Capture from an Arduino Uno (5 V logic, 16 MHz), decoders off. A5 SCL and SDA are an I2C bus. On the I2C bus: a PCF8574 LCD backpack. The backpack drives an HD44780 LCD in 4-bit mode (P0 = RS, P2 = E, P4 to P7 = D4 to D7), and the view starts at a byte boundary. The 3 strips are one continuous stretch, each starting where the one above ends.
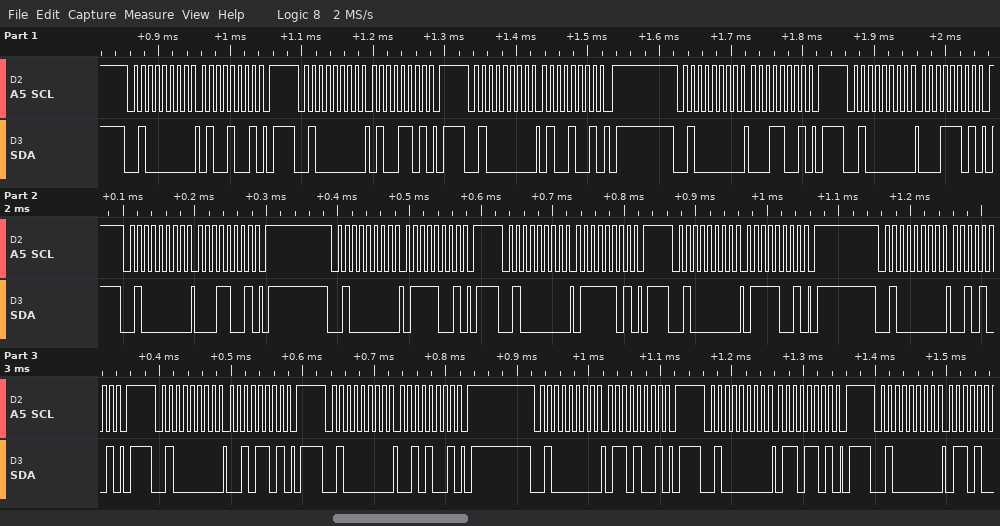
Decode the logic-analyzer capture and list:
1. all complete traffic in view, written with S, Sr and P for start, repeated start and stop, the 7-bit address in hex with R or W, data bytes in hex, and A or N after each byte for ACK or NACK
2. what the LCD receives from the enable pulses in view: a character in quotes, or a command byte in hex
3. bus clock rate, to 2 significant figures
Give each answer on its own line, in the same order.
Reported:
S 20W A 49 A P S 20W A 4D A P S 20W A 49 A P S 20W A 19 A P S 20W A 1D A P S 20W A 19 A P S 20W A 79 A P S 20W A 7D A P S 20W A 79 A P S 20W A 29 A P S 20W A 2D A P S 20W A 29 A P S 20W A 69 A P S 20W A 6D A P S 20W A
'A' 'r'
100 kHz
